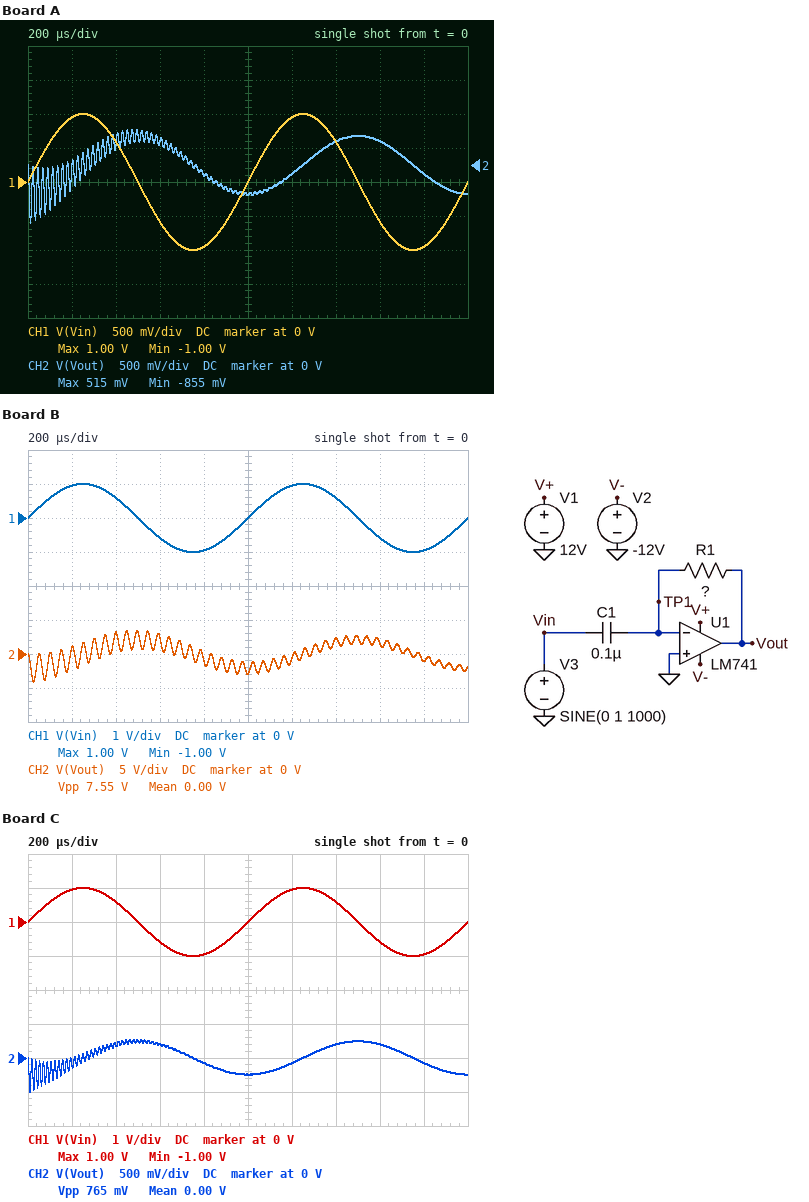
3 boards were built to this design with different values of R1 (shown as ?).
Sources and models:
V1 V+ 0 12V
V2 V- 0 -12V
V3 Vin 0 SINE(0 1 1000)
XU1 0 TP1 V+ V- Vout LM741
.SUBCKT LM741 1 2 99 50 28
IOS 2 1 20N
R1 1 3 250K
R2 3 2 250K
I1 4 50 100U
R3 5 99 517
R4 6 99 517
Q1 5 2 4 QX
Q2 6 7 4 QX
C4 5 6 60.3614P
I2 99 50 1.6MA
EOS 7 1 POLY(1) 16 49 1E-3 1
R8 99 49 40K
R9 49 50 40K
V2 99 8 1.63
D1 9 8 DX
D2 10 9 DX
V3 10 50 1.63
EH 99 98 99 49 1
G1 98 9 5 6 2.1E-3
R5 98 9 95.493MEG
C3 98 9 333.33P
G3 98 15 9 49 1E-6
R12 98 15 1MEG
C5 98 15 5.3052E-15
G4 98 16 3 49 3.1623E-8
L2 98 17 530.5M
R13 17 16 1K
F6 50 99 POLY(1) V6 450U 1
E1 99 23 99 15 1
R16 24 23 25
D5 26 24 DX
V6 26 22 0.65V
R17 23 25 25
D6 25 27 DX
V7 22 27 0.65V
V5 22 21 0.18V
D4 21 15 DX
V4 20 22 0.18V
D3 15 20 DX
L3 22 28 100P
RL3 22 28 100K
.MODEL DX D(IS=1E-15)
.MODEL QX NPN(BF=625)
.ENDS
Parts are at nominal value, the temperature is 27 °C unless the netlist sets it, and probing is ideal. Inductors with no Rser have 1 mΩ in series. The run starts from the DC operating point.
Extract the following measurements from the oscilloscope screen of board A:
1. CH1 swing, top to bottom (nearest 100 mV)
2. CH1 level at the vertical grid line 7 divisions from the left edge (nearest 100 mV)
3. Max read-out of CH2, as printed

2.0 V
600 mV
515 mV
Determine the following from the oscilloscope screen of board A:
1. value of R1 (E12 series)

680 Ω
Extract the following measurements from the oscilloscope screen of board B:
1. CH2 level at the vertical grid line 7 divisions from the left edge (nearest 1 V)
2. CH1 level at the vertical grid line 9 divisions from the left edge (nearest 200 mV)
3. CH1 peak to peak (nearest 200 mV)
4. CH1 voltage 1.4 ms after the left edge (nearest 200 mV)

2 V
-1.0 V
2.0 V
600 mV
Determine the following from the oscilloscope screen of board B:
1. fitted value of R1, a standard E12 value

3.3 kΩ
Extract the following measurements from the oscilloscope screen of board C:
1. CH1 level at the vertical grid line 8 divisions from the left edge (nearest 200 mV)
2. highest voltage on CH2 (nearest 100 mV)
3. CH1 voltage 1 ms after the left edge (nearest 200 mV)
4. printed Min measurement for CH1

-600 mV
300 mV
0 V
-1.00 V
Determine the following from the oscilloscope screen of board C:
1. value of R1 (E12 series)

390 Ω
